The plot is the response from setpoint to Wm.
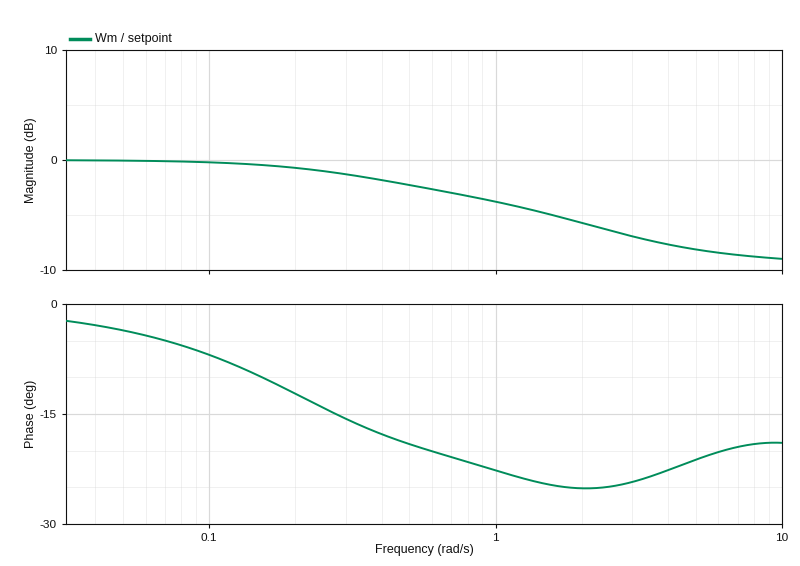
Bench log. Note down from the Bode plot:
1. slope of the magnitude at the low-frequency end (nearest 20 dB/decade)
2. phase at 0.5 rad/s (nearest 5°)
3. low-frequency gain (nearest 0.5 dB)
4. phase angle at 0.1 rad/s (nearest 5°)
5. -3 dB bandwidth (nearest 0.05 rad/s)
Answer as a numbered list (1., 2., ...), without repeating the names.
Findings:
1. 0 dB/decade
2. -20°
3. 0.0 dB
4. -5°
5. 0.70 rad/s
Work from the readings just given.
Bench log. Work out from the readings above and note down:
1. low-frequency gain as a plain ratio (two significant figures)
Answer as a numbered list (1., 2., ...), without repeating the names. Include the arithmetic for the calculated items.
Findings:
1. 10^(0 / 20) = 1.0
